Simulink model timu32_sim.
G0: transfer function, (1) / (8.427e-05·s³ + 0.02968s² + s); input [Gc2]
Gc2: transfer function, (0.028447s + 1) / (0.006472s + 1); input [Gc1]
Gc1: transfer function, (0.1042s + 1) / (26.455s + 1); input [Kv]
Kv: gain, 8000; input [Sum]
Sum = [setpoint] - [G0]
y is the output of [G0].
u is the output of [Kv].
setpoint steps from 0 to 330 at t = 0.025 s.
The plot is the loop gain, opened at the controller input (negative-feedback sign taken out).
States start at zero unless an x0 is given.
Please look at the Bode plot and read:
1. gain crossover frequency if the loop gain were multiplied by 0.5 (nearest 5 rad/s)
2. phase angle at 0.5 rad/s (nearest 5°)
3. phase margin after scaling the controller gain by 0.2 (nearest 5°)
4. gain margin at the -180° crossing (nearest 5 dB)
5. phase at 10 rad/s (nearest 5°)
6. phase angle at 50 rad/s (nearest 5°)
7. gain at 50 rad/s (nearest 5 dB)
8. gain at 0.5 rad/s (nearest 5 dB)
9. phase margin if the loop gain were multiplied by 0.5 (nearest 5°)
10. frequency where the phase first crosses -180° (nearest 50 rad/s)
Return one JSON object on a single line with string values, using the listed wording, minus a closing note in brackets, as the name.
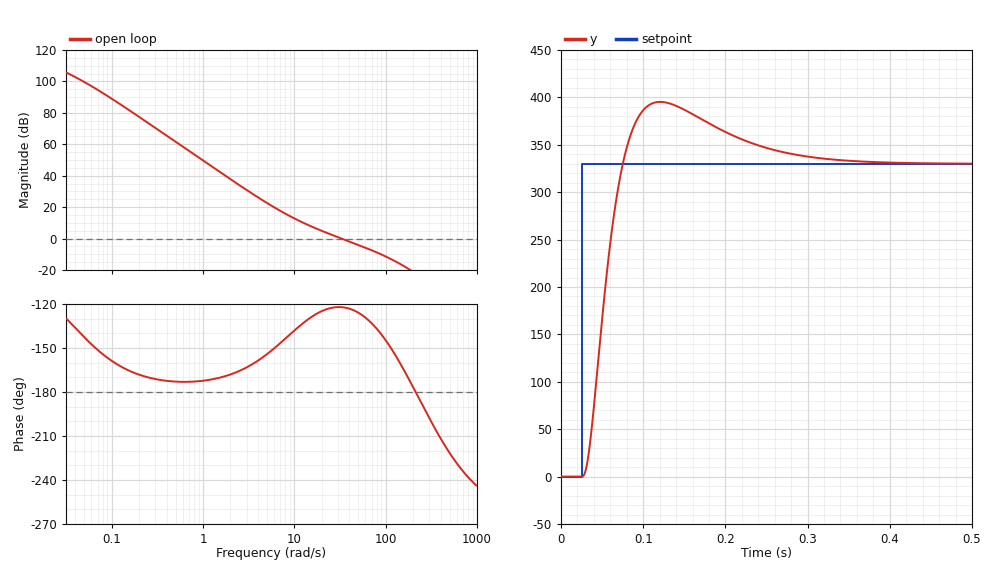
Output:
{"gain crossover frequency if the loop gain were multiplied by 0.5": "20 rad/s", "phase angle at 0.5 rad/s": "-175°", "phase margin after scaling the controller gain by 0.2": "40°", "gain margin at the -180° crossing": "20 dB", "phase at 10 rad/s": "-140°", "phase angle at 50 rad/s": "-125°", "gain at 50 rad/s": "-5 dB", "gain at 0.5 rad/s": "60 dB", "phase margin if the loop gain were multiplied by 0.5": "55°", "frequency where the phase first crosses -180°": "200 rad/s"}
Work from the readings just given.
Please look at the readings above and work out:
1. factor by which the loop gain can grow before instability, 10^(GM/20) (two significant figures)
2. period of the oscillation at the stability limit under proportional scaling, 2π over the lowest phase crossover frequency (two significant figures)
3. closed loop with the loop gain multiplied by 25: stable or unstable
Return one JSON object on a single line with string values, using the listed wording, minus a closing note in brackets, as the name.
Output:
{"factor by which the loop gain can grow before instability, 10^(GM/20)": "10", "period of the oscillation at the stability limit under proportional scaling, 2π over the lowest phase crossover frequency": "0.031 s", "closed loop with the loop gain multiplied by 25: stable or unstable": "unstable"}
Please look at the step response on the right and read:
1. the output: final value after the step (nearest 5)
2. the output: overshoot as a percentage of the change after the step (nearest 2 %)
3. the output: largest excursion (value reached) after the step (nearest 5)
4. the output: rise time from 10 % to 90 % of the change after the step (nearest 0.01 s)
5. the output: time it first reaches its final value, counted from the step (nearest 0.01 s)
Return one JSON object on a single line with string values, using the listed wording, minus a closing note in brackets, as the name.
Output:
{"the output: final value after the step": "330", "the output: overshoot as a percentage of the change after the step": "20 %", "the output: largest excursion (value reached) after the step": "395", "the output: rise time from 10 % to 90 % of the change after the step": "0.03 s", "the output: time it first reaches its final value, counted from the step": "0.05 s"}
